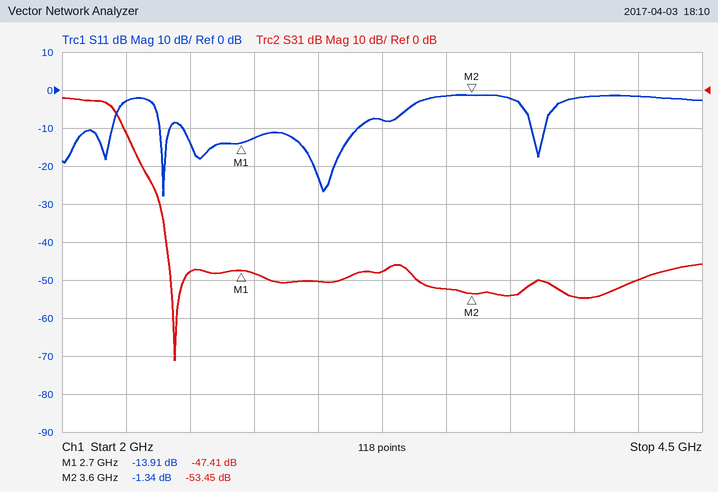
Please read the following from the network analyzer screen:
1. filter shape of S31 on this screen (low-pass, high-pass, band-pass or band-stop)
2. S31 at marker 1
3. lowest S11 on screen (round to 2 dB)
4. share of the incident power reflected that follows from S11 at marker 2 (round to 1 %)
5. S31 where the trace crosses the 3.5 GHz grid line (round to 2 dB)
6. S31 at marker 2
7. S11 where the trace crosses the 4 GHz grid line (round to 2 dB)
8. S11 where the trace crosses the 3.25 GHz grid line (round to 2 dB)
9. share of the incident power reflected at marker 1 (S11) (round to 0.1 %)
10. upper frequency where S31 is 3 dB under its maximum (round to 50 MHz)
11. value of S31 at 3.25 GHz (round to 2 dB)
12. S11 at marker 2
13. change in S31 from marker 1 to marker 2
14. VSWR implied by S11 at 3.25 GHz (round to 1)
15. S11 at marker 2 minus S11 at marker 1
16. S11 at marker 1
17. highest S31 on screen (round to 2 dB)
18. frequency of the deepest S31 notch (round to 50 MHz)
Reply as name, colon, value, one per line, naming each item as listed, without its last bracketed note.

filter shape of S31 on this screen: low-pass
S31 at marker 1: -47.41 dB
lowest S11 on screen: -28 dB
share of the incident power reflected that follows from S11 at marker 2: 73 %
S31 where the trace crosses the 3.5 GHz grid line: -52 dB
S31 at marker 2: -53.45 dB
S11 where the trace crosses the 4 GHz grid line: -2 dB
S11 where the trace crosses the 3.25 GHz grid line: -8 dB
share of the incident power reflected at marker 1 (S11): 4.1 %
upper frequency where S31 is 3 dB under its maximum: 2.20 GHz
value of S31 at 3.25 GHz: -48 dB
S11 at marker 2: -1.34 dB
change in S31 from marker 1 to marker 2: -6.04 dB
VSWR implied by S11 at 3.25 GHz: 2
S11 at marker 2 minus S11 at marker 1: 12.57 dB
S11 at marker 1: -13.91 dB
highest S31 on screen: -2 dB
frequency of the deepest S31 notch: 2.45 GHz
